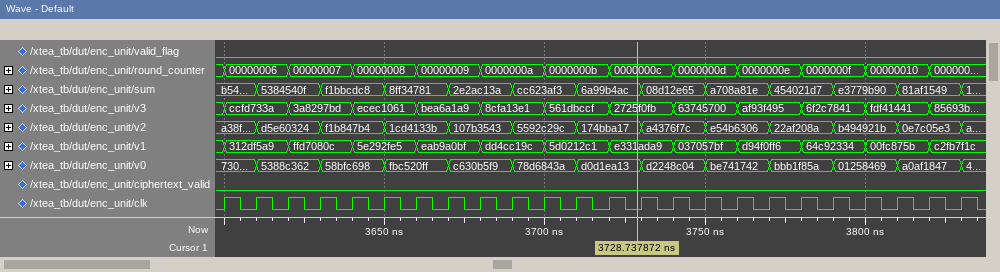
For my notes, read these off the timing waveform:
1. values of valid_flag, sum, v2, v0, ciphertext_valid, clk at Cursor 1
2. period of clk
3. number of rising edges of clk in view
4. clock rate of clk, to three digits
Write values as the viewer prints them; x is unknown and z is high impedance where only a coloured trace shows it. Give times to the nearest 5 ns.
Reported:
valid_flag=0, sum=6a99b4ac, v2=174bba17, v0=d0d1ea13, ciphertext_valid=0, clk=0
10 ns
24
100 MHz
